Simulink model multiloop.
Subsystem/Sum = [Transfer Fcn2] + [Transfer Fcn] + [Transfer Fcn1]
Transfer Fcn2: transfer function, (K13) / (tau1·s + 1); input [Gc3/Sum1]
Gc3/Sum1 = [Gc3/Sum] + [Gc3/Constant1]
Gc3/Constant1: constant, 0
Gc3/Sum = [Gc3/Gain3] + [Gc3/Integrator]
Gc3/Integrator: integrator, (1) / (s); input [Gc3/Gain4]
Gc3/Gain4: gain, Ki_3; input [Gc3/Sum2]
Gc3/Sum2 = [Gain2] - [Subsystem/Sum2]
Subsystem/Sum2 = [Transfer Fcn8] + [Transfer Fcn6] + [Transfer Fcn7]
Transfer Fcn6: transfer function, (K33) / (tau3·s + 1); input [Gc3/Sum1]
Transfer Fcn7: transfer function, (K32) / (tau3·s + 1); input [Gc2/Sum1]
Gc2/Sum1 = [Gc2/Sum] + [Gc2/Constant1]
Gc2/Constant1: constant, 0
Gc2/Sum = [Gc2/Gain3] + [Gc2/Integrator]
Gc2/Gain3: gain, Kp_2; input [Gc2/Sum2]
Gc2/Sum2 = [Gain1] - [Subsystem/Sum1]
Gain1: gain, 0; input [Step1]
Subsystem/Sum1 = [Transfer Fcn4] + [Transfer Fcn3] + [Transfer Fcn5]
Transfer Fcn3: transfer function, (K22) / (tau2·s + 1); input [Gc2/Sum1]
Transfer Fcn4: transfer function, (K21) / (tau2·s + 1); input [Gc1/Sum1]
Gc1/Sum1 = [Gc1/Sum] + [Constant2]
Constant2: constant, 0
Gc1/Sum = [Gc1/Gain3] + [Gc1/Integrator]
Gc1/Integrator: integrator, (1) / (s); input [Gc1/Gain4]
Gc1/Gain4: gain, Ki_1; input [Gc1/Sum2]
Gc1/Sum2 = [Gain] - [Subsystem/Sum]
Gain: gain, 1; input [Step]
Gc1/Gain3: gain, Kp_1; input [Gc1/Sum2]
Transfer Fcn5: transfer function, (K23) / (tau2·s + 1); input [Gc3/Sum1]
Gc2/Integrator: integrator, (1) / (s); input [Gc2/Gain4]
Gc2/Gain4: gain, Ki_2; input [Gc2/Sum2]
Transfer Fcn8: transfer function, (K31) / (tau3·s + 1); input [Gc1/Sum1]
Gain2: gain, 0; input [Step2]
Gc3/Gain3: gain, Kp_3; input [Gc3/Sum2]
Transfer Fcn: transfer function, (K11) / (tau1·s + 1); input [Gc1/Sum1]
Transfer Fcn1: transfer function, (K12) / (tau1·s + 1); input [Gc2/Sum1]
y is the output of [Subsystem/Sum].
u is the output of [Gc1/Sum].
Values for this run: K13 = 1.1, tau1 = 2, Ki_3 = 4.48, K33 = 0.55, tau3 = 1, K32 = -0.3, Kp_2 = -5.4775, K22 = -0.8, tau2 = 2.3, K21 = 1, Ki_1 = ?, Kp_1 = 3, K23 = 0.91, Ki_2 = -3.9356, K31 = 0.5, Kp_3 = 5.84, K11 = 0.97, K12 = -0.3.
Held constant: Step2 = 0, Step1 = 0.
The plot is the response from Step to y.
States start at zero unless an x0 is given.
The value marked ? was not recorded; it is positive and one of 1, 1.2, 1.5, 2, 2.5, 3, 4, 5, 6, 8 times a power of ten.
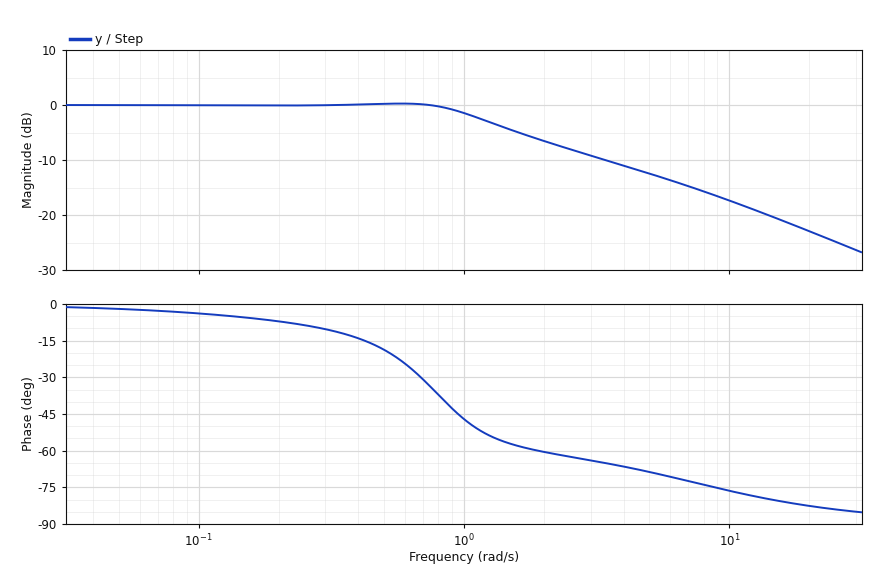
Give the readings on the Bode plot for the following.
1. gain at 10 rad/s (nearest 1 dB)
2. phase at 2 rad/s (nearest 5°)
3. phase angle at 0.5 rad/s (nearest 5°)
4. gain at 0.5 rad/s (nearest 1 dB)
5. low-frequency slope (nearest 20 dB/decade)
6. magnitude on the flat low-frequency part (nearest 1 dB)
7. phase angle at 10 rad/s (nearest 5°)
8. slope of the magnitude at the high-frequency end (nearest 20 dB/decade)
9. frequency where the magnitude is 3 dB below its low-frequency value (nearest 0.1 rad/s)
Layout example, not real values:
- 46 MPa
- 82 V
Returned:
- -17 dB
- -60°
- -20°
- 0 dB
- 0 dB/decade
- 0 dB
- -75°
- -20 dB/decade
- 1.2 rad/s
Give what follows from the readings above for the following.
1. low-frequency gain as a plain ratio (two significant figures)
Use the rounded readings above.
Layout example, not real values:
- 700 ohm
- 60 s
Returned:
- 1.0
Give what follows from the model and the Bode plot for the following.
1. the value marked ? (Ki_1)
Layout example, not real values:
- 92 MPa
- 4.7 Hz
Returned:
- 10
